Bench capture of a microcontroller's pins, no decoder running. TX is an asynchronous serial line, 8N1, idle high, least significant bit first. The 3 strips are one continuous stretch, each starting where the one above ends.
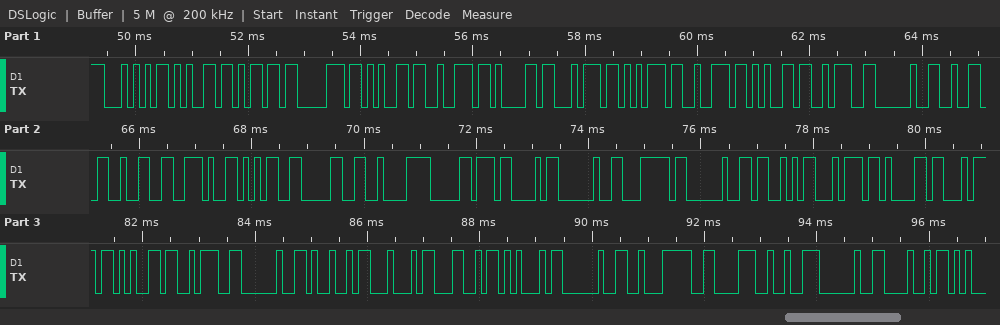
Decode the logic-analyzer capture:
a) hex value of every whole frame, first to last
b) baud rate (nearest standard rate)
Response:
54 65 6D 70 65 72 61 74 75 72 65 3A 20 32 32 2E 35 30 C2 B0 43 20 7C 20 53 74 61 74 65 3A 20 49 44 4C 45 20 E2 86 92 20 48
9600 baud
